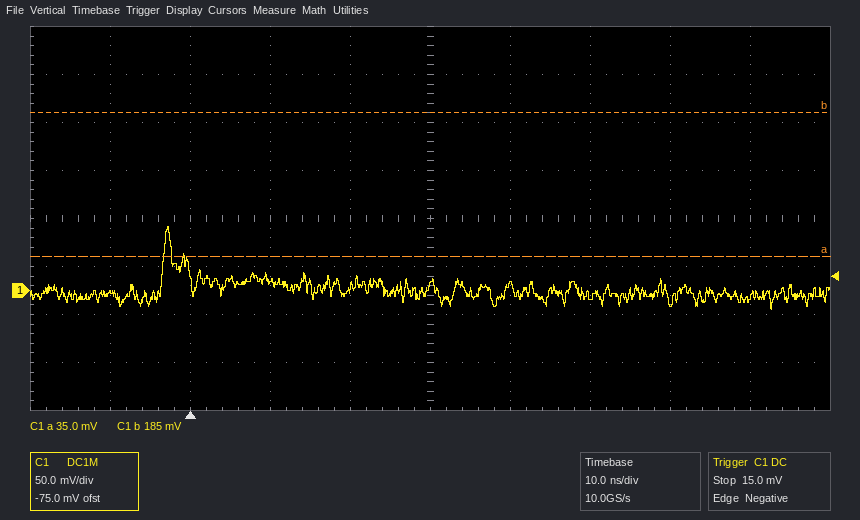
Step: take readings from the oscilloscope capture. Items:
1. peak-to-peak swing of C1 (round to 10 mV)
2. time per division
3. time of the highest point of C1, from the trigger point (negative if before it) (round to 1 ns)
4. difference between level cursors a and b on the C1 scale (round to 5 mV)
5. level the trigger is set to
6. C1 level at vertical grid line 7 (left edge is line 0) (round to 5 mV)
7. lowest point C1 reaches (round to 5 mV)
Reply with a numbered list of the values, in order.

1. 90 mV
2. 10 ns
3. -3 ns
4. 150 mV
5. 15.0 mV
6. -5 mV
7. -20 mV
